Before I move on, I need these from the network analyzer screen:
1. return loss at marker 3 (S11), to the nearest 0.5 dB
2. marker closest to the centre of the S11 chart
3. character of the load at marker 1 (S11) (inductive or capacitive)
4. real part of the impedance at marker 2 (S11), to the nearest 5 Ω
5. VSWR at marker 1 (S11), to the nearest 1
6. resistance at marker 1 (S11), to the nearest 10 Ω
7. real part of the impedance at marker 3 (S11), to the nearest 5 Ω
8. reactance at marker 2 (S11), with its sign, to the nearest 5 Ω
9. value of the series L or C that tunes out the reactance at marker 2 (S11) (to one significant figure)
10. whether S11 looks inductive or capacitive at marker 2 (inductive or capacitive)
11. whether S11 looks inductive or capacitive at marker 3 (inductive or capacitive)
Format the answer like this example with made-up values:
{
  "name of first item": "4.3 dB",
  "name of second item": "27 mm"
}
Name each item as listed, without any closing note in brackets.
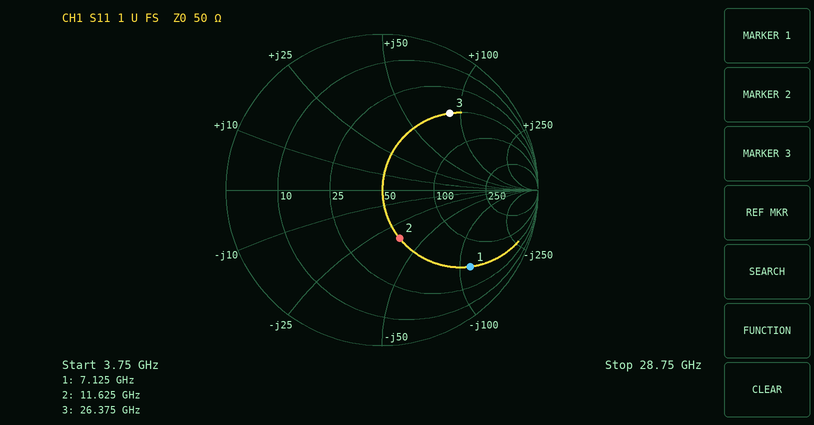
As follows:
{
  "return loss at marker 3 (S11), to the nearest 0.5 dB": "3.5 dB",
  "marker closest to the centre of the S11 chart": "marker 2",
  "character of the load at marker 1 (S11)": "capacitive",
  "real part of the impedance at marker 2 (S11), to the nearest 5 Ω": "50 Ω",
  "VSWR at marker 1 (S11), to the nearest 1": "7",
  "resistance at marker 1 (S11), to the nearest 10 Ω": "50 Ω",
  "real part of the impedance at marker 3 (S11), to the nearest 5 Ω": "50 Ω",
  "reactance at marker 2 (S11), with its sign, to the nearest 5 Ω": "-35 Ω",
  "value of the series L or C that tunes out the reactance at marker 2 (S11)": "500 pH",
  "whether S11 looks inductive or capacitive at marker 2": "capacitive",
  "whether S11 looks inductive or capacitive at marker 3": "inductive"
}
